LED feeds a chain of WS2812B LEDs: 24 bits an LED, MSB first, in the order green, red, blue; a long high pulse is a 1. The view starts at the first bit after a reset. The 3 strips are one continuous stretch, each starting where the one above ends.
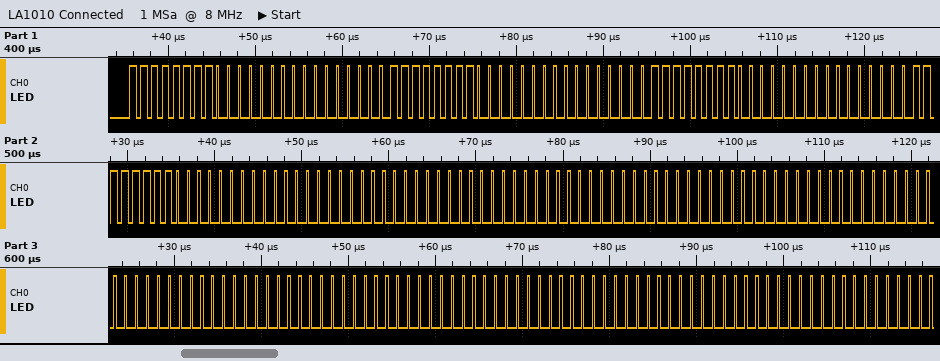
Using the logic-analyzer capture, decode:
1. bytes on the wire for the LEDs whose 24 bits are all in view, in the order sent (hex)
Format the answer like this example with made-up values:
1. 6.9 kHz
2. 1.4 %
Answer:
1. FF 00 00 FF 00 00 FF 00 00 FF 00 00 00 00 00 00 00 00 00 00 00 00 00 00 00 00 00
